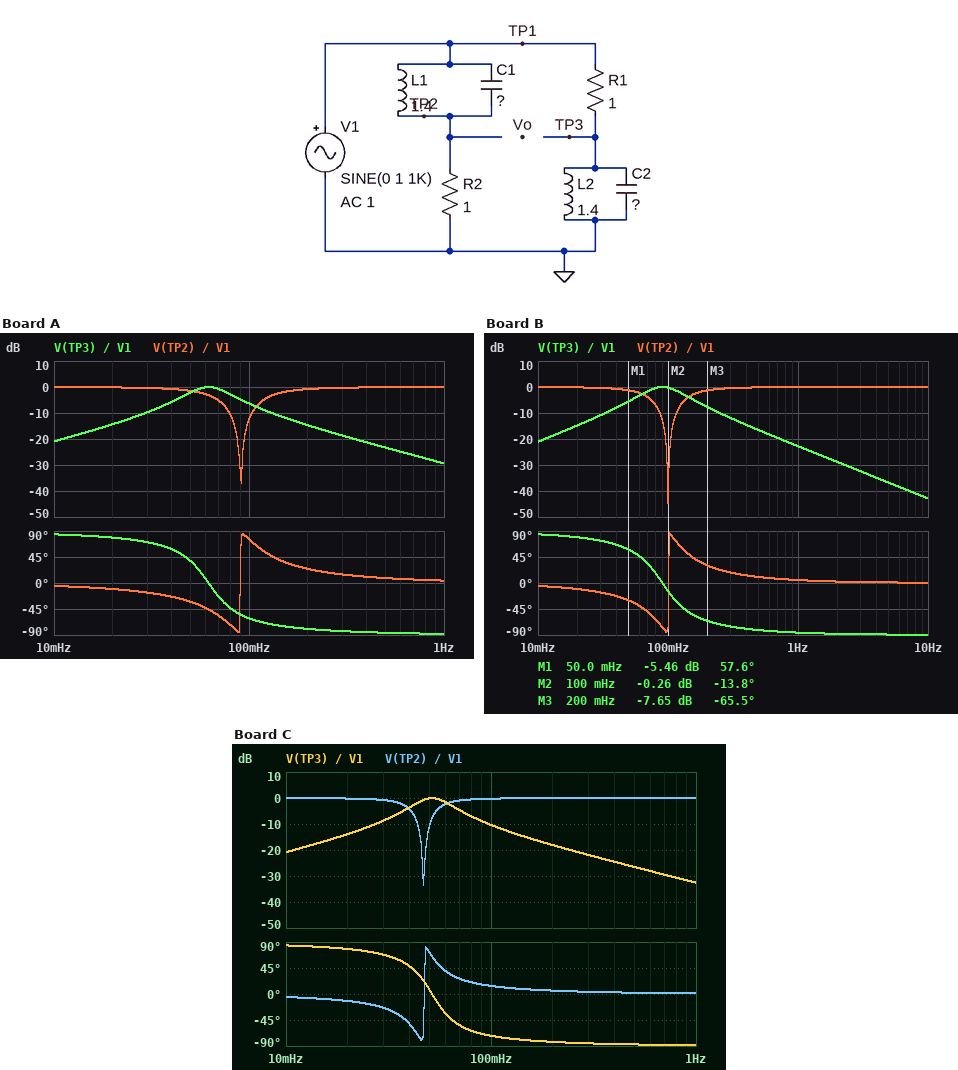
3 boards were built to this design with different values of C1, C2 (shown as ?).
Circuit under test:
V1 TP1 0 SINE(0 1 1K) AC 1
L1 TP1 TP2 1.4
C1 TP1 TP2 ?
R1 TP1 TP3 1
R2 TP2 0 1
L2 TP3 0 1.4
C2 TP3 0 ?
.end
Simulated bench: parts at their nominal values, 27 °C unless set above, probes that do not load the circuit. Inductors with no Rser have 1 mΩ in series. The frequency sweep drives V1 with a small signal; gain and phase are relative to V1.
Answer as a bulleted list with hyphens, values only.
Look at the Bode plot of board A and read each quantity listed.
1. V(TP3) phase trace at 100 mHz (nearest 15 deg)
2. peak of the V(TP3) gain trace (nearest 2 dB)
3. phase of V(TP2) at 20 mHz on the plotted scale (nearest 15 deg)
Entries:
- -60 deg
- 0 dB
- -15 deg
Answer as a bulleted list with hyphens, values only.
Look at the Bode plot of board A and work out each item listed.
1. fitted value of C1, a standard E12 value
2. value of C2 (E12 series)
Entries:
- 2.2 F
- 4.7 F
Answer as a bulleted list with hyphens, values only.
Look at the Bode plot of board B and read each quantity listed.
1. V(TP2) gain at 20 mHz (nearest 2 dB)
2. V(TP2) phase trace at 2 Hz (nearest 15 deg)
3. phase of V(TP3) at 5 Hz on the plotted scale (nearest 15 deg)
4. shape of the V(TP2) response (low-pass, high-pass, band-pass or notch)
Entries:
- 0 dB
- 0 deg
- -90 deg
- notch
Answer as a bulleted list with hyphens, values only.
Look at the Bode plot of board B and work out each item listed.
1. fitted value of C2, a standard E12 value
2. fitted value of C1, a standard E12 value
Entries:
- 2.2 F
- 1.8 F
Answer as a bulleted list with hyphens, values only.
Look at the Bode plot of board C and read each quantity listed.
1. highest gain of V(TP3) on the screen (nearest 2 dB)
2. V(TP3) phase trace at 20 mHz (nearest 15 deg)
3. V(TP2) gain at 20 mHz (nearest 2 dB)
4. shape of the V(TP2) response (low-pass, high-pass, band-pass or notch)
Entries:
- 0 dB
- 75 deg
- 0 dB
- notch
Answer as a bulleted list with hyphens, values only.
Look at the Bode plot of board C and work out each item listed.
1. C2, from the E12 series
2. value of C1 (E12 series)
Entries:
- 6.8 F
- 8.2 F
